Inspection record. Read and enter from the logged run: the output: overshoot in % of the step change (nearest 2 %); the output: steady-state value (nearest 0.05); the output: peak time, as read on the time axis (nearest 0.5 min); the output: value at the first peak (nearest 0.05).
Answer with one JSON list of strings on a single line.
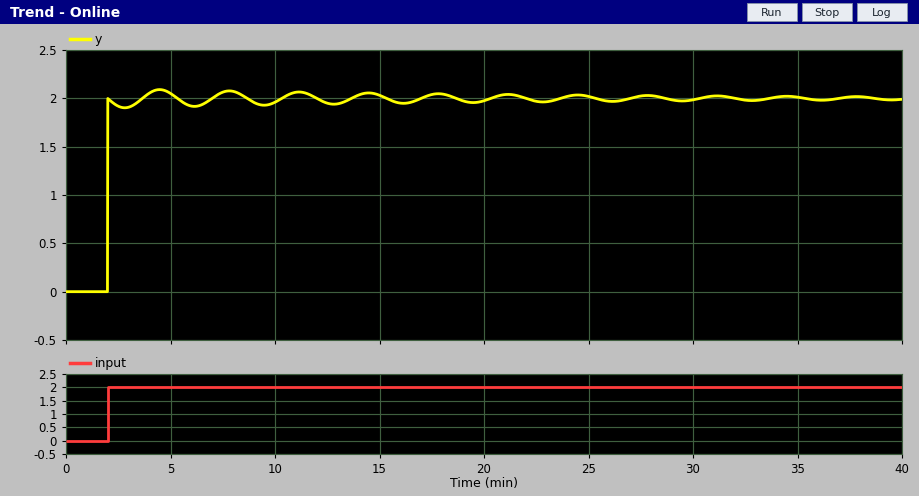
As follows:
["4 %", "2.00", "4.5 min", "2.10"]
